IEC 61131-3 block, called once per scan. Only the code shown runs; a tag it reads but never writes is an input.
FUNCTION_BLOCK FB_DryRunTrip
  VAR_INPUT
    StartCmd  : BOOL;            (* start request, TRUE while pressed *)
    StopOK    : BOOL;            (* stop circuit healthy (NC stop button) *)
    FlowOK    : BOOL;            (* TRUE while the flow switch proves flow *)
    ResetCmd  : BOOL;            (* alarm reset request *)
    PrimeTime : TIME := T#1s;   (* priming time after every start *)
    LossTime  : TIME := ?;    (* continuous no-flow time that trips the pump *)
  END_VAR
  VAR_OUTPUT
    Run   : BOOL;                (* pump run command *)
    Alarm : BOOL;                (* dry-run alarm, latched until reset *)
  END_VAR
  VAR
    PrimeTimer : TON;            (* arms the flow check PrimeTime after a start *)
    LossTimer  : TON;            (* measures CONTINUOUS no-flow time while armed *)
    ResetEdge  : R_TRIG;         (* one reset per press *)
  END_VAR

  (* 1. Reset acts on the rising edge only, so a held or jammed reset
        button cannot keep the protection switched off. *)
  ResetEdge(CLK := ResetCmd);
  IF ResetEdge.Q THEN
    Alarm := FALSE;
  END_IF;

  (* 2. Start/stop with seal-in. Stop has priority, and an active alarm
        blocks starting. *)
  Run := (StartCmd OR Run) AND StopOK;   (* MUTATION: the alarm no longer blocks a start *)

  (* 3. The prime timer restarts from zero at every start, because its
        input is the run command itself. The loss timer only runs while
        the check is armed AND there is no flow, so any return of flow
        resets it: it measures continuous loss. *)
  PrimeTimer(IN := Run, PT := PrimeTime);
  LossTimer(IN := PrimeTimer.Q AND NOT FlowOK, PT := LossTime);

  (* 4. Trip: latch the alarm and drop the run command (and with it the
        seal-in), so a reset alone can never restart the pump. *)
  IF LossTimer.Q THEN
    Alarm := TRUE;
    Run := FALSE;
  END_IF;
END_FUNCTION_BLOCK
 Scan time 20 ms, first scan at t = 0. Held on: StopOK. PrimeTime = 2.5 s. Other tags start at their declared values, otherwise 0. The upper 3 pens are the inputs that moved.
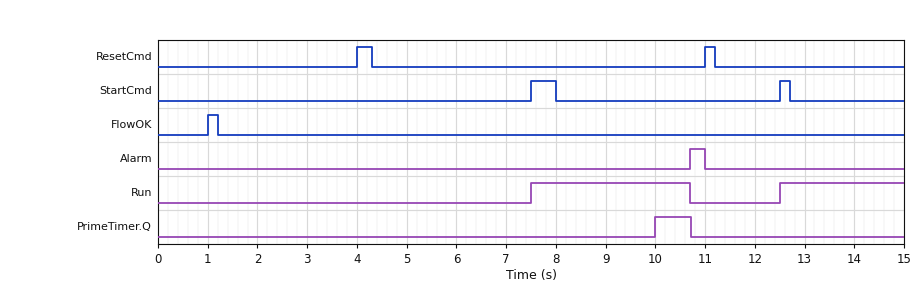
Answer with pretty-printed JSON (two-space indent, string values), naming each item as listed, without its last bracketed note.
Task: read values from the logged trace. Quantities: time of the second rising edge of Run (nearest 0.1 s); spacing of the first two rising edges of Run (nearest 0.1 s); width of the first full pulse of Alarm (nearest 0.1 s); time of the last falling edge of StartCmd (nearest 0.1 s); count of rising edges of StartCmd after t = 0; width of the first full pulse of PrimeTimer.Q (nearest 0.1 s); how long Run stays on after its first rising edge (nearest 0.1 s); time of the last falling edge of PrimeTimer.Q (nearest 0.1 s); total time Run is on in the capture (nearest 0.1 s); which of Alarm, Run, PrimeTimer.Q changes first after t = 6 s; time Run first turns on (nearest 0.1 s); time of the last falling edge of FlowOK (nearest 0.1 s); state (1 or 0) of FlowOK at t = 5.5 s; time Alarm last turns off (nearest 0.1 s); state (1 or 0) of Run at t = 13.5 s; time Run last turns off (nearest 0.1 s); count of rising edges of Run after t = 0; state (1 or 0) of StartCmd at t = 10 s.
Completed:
{
  "time of the second rising edge of Run": "12.5 s",
  "spacing of the first two rising edges of Run": "5.0 s",
  "width of the first full pulse of Alarm": "0.3 s",
  "time of the last falling edge of StartCmd": "12.7 s",
  "count of rising edges of StartCmd after t = 0": "2",
  "width of the first full pulse of PrimeTimer.Q": "0.7 s",
  "how long Run stays on after its first rising edge": "3.2 s",
  "time of the last falling edge of PrimeTimer.Q": "10.7 s",
  "total time Run is on in the capture": "5.7 s",
  "which of Alarm, Run, PrimeTimer.Q changes first after t = 6 s": "Run",
  "time Run first turns on": "7.5 s",
  "time of the last falling edge of FlowOK": "1.2 s",
  "state (1 or 0) of FlowOK at t = 5.5 s": "0",
  "time Alarm last turns off": "11.0 s",
  "state (1 or 0) of Run at t = 13.5 s": "1",
  "time Run last turns off": "10.7 s",
  "count of rising edges of Run after t = 0": "2",
  "state (1 or 0) of StartCmd at t = 10 s": "0"
}
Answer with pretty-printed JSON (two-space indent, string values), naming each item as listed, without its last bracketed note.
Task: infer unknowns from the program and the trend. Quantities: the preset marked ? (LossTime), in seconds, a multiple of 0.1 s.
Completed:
{
  "the preset marked ? (LossTime), in seconds, a multiple of 0.1 s": "0.7 s"
}
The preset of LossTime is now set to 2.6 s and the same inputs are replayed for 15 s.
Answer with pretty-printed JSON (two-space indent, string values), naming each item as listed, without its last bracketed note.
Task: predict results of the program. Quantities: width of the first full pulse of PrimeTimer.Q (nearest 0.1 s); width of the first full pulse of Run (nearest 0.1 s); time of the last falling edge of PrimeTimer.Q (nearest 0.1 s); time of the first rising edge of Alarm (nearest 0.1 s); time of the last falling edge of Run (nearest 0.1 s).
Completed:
{
  "width of the first full pulse of PrimeTimer.Q": "2.7 s",
  "width of the first full pulse of Run": "5.1 s",
  "time of the last falling edge of PrimeTimer.Q": "12.7 s",
  "time of the first rising edge of Alarm": "12.6 s",
  "time of the last falling edge of Run": "12.6 s"
}
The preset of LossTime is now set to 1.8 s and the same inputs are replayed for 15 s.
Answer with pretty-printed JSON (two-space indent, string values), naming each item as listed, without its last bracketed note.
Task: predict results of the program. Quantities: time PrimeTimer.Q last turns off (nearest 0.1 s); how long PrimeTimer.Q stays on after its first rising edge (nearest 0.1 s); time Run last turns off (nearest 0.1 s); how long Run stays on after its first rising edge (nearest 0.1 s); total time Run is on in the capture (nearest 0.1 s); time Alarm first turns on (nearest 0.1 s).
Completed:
{
  "time PrimeTimer.Q last turns off": "11.8 s",
  "how long PrimeTimer.Q stays on after its first rising edge": "1.8 s",
  "time Run last turns off": "11.8 s",
  "how long Run stays on after its first rising edge": "4.3 s",
  "total time Run is on in the capture": "6.8 s",
  "time Alarm first turns on": "11.8 s"
}
